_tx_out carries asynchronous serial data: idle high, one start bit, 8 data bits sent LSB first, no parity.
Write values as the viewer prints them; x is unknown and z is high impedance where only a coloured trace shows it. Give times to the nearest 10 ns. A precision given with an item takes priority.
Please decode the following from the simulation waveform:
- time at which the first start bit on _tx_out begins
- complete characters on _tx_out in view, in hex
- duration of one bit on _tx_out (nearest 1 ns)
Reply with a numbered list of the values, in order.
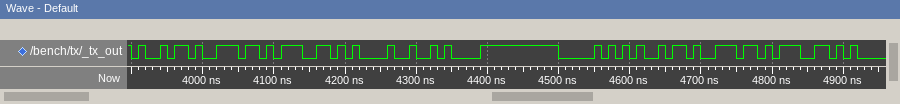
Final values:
1. 3900 ns
2. 69, 6E, 67, 21, 0A, 50, 69, 6E, 67
3. 10 ns
